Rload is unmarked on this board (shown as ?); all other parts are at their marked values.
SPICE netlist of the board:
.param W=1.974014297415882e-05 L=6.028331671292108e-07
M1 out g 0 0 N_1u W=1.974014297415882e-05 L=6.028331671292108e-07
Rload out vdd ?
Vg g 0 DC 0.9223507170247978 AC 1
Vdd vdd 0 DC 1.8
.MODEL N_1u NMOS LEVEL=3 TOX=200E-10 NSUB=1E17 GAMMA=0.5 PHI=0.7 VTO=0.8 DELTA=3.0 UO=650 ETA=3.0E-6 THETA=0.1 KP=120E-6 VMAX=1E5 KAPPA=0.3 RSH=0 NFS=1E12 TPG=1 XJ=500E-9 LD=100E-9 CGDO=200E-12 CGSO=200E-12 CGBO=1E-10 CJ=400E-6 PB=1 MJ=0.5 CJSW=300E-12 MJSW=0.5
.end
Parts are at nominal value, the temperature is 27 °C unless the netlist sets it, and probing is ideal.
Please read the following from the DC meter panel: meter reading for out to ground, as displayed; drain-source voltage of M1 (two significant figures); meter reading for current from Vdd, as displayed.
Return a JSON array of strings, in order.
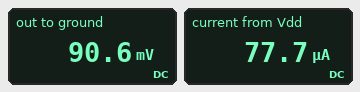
["90.6 mV", "91 mV", "77.7 µA"]
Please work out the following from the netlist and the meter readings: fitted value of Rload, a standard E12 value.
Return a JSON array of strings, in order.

["22 kΩ"]
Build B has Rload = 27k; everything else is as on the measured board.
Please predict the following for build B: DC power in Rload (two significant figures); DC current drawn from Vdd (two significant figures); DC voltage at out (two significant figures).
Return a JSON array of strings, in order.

["110 µW", "64 µA", "67 mV"]
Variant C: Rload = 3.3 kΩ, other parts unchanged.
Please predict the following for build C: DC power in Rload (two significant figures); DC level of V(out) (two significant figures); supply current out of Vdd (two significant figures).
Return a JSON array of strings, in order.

["42 µW", "1.4 V", "110 µA"]
